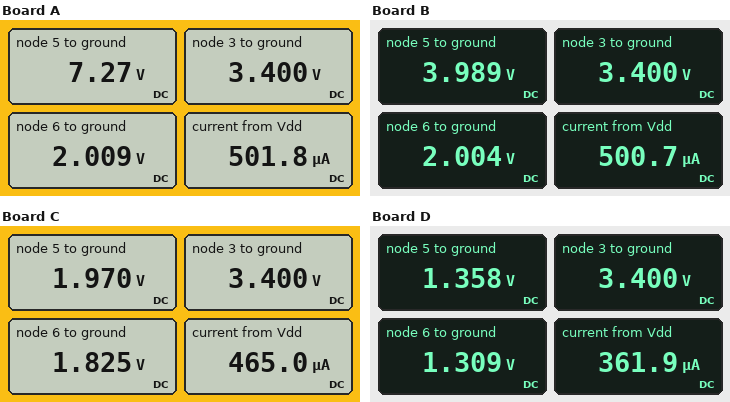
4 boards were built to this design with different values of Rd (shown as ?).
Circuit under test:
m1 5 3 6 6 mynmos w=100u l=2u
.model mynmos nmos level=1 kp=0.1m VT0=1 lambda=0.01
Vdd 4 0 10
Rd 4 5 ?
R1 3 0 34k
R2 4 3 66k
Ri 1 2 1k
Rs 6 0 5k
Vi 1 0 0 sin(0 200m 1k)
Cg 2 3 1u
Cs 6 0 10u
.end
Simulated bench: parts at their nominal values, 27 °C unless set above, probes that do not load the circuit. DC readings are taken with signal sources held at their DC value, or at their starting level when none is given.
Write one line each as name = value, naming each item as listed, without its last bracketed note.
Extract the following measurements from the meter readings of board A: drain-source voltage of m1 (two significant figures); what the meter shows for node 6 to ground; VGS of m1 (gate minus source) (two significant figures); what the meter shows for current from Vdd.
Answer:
drain-source voltage of m1 = 5.3 V
what the meter shows for node 6 to ground = 2.009 V
VGS of m1 (gate minus source) = 1.4 V
what the meter shows for current from Vdd = 501.8 µA
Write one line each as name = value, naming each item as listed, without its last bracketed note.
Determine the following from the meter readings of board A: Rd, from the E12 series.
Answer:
Rd, from the E12 series = 6.8 kΩ
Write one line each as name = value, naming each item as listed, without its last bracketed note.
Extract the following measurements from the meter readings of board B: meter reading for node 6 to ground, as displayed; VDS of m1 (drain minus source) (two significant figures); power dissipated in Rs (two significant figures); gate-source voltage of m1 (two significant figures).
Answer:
meter reading for node 6 to ground, as displayed = 2.004 V
VDS of m1 (drain minus source) = 2.0 V
power dissipated in Rs = 800 µW
gate-source voltage of m1 = 1.4 V
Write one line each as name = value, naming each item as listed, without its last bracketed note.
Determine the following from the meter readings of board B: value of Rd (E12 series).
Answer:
value of Rd = 15 kΩ
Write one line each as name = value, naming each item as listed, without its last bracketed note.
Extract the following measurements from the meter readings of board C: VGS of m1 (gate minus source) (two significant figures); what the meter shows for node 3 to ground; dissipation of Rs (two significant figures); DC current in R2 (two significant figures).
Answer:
VGS of m1 (gate minus source) = 1.6 V
what the meter shows for node 3 to ground = 3.400 V
dissipation of Rs = 670 µW
DC current in R2 = 100 µA
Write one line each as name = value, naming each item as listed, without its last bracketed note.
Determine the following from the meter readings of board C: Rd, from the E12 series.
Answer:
Rd, from the E12 series = 22 kΩ
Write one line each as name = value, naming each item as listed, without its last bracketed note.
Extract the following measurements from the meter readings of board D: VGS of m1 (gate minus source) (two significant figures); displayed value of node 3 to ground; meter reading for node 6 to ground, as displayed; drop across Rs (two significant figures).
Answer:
VGS of m1 (gate minus source) = 2.1 V
displayed value of node 3 to ground = 3.400 V
meter reading for node 6 to ground, as displayed = 1.309 V
drop across Rs = 1.3 V
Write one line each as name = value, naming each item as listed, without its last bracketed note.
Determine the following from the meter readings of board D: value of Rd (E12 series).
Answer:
value of Rd = 33 kΩ
